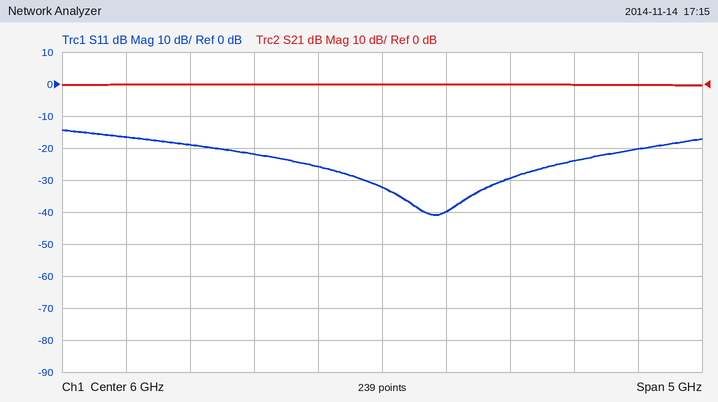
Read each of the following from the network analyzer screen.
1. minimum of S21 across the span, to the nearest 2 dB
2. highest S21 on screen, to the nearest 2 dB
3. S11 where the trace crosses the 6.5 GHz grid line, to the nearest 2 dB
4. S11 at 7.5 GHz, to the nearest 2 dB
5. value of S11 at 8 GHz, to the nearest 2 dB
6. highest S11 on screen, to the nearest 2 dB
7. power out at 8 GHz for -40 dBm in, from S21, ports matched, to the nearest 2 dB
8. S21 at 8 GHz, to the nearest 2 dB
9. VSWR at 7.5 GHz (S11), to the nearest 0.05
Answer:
0 dB
0 dB
-40 dB
-24 dB
-20 dB
-14 dB
-40 dBm
0 dB
1.15
